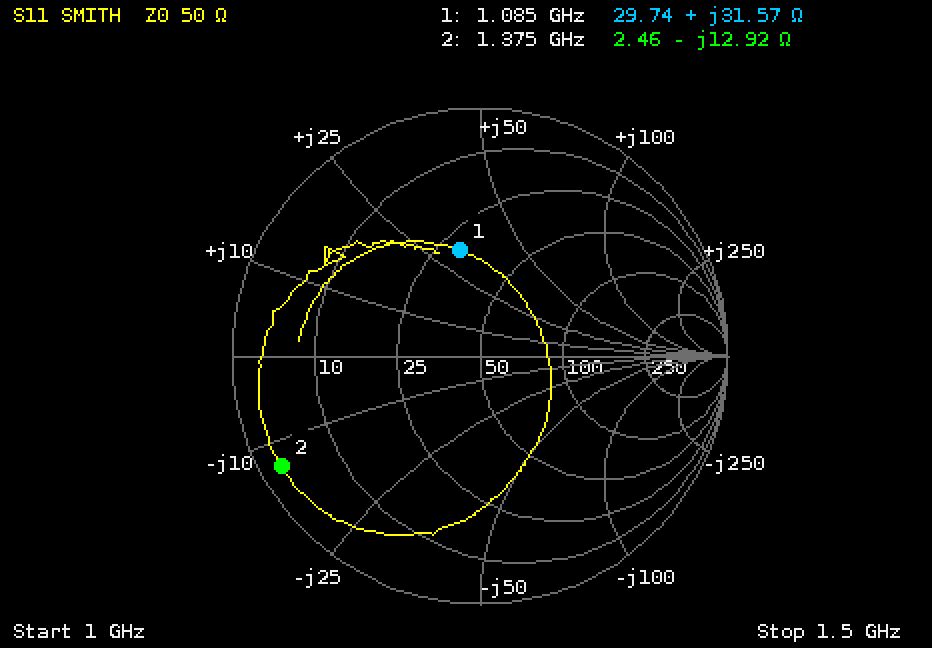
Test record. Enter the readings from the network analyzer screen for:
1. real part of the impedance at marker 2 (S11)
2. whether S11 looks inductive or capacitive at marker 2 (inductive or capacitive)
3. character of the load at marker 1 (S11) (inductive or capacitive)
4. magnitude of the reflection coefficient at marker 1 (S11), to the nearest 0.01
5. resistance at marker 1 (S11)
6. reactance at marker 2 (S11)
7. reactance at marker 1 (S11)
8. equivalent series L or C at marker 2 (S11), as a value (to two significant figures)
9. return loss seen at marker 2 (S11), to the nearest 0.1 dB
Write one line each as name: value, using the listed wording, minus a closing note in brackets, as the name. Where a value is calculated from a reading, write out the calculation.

real part of the impedance at marker 2: 2.46 Ω
whether S11 looks inductive or capacitive at marker 2: capacitive
character of the load at marker 1 (S11): inductive
magnitude of the reflection coefficient at marker 1 (S11), to the nearest 0.01: 0.44
resistance at marker 1: 29.74 Ω
reactance at marker 2: -12.92 Ω
reactance at marker 1: +31.57 Ω
equivalent series L or C at marker 2 (S11), as a value: C = 1/(2π × 1.375 GHz × 12.92 Ω) ≈ 9.0 pF
return loss seen at marker 2 (S11), to the nearest 0.1 dB: 0.8 dB
